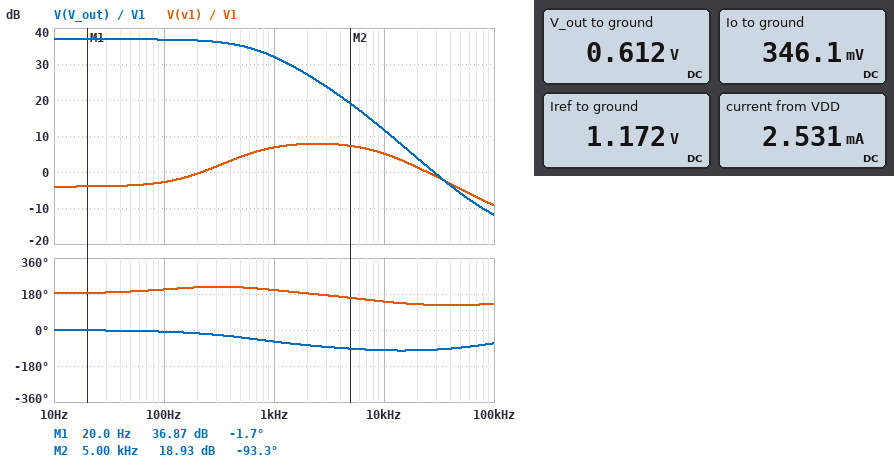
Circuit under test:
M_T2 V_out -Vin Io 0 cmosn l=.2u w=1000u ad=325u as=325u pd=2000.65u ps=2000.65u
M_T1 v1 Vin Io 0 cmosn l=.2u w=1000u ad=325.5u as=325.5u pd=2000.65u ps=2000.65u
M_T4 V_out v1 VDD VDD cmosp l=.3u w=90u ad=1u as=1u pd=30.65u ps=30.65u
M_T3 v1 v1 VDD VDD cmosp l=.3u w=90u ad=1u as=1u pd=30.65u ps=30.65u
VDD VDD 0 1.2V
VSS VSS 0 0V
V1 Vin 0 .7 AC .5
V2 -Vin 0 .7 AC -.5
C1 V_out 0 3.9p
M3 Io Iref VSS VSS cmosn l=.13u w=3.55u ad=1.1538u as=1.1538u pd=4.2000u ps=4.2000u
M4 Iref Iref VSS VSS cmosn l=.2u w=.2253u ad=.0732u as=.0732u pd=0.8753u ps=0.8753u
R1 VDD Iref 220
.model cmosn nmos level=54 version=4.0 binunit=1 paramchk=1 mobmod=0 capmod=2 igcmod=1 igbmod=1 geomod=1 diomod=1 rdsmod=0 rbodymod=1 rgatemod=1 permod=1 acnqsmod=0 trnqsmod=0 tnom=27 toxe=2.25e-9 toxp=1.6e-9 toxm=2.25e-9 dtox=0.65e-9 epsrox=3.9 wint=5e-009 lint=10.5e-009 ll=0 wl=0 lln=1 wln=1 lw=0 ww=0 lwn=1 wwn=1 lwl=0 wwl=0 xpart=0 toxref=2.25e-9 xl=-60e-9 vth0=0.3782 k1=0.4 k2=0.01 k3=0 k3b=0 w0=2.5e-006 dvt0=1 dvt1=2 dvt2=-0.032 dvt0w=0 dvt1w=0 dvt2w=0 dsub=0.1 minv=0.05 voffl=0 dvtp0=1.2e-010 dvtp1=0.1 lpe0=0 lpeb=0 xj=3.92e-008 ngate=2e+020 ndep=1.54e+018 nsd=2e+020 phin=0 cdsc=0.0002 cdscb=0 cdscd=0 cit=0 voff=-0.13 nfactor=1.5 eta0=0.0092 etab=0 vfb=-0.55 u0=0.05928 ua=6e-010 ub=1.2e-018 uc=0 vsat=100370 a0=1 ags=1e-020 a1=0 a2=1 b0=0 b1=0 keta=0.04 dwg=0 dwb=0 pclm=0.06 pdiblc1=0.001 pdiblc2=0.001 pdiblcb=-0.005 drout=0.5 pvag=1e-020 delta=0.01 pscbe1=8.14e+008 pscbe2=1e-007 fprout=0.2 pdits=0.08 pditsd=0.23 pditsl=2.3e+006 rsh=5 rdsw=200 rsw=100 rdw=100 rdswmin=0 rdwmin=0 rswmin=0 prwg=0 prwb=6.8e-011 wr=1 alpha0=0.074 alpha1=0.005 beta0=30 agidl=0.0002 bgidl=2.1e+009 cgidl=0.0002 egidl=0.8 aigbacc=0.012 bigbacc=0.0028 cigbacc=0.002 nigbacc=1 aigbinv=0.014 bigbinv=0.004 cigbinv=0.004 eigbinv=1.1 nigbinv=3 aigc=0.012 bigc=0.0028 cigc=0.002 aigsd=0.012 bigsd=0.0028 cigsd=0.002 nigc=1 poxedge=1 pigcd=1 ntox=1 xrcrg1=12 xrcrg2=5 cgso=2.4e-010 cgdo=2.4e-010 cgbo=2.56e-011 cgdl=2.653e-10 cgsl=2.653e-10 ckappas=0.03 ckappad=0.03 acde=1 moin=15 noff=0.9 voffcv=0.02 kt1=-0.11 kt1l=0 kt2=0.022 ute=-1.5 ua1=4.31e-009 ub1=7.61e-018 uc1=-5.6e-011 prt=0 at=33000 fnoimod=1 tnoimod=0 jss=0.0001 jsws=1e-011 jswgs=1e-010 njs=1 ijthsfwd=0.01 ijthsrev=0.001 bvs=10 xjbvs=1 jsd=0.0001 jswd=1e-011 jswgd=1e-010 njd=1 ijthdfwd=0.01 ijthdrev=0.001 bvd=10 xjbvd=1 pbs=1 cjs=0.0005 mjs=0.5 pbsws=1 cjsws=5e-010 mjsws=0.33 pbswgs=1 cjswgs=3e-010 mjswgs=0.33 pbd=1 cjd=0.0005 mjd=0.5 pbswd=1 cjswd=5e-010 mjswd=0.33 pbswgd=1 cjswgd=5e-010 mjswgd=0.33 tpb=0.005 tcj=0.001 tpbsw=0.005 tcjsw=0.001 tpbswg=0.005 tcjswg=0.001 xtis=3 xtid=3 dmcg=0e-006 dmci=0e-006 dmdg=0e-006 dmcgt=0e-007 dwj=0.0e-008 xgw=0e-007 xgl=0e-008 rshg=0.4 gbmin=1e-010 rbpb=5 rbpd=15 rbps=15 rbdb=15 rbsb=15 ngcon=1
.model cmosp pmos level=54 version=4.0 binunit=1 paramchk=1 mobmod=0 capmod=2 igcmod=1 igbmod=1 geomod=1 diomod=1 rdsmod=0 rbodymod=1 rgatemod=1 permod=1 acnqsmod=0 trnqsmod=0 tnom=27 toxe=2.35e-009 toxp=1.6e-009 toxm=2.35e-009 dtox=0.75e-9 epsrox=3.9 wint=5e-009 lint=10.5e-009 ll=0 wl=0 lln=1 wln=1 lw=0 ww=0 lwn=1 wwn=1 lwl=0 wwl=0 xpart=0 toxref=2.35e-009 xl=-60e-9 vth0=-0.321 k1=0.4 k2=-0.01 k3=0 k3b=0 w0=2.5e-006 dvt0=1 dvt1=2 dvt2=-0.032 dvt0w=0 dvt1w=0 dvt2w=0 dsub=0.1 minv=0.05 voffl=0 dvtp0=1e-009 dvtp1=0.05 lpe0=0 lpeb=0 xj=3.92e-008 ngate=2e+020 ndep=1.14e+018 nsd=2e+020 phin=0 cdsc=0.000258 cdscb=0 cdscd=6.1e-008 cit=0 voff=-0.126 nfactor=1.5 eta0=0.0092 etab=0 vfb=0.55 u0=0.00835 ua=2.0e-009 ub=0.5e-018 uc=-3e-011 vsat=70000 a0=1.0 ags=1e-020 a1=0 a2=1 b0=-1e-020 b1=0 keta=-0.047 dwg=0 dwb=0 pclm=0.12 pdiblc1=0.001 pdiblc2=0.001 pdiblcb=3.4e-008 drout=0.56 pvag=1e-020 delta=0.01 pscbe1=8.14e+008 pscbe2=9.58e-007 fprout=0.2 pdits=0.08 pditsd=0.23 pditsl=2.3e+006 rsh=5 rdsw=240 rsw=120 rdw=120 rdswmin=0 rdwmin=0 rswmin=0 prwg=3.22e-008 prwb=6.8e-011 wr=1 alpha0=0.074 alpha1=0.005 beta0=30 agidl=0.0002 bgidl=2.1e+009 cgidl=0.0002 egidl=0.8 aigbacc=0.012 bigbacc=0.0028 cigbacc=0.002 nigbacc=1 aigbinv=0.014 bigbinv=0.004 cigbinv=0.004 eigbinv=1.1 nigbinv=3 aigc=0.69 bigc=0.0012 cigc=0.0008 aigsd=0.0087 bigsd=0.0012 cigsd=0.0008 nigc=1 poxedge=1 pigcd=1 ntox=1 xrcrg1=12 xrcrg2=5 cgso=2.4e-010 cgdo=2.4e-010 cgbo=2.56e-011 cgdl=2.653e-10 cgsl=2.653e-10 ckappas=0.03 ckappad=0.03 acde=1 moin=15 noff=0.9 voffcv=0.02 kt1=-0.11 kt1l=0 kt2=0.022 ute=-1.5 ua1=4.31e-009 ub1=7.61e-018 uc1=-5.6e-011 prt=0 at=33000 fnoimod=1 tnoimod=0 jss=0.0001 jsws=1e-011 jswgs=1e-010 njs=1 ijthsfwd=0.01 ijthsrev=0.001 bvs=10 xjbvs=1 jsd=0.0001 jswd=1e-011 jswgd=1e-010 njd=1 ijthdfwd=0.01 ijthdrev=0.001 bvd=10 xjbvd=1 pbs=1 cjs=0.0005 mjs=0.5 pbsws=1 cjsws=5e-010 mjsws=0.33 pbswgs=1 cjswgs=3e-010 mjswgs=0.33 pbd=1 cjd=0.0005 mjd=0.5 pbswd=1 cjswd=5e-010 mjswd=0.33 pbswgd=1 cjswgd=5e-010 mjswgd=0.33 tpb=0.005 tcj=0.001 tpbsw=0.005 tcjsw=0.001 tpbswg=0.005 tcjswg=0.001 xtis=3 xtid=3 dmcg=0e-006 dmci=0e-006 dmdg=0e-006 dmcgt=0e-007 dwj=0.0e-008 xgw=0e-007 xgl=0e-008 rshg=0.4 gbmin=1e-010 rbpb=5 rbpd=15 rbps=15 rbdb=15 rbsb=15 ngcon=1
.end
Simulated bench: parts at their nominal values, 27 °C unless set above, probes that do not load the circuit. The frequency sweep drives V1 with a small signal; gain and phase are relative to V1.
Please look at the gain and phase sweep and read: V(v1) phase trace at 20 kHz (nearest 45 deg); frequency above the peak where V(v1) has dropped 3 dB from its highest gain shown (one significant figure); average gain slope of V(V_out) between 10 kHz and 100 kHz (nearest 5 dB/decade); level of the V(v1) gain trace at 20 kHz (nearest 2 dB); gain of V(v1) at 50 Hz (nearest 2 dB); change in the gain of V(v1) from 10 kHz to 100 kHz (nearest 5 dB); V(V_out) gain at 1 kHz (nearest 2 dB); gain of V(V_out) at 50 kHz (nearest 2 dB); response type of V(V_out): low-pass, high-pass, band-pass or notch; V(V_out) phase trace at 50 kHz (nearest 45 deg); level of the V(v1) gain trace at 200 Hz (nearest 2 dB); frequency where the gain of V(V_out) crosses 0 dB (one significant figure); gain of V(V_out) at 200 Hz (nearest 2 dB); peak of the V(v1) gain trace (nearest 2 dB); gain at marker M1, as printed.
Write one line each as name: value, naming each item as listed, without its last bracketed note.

V(v1) phase trace at 20 kHz: 135 deg
frequency above the peak where V(v1) has dropped 3 dB from its highest gain shown: 10 kHz
average gain slope of V(V_out) between 10 kHz and 100 kHz: -25 dB/decade
level of the V(v1) gain trace at 20 kHz: 2 dB
gain of V(v1) at 50 Hz: -4 dB
change in the gain of V(v1) from 10 kHz to 100 kHz: -15 dB
V(V_out) gain at 1 kHz: 32 dB
gain of V(V_out) at 50 kHz: -6 dB
response type of V(V_out): low-pass, high-pass, band-pass or notch: low-pass
V(V_out) phase trace at 50 kHz: -90 deg
level of the V(v1) gain trace at 200 Hz: 0 dB
frequency where the gain of V(V_out) crosses 0 dB: 30 kHz
gain of V(V_out) at 200 Hz: 36 dB
peak of the V(v1) gain trace: 8 dB
gain at marker M1, as printed: 36.87 dB
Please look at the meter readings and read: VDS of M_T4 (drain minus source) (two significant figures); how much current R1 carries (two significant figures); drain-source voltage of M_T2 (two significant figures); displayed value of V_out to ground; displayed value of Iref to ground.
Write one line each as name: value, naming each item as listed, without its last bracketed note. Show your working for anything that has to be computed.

VDS of M_T4 (drain minus source): 612 mV - 1.2 V = -590 mV
how much current R1 carries: (1.2 V - 1.172 V) / 220 Ω = 130 µA
drain-source voltage of M_T2: 612 mV - 346.1 mV = 270 mV
displayed value of V_out to ground: 0.612 V
displayed value of Iref to ground: 1.172 V
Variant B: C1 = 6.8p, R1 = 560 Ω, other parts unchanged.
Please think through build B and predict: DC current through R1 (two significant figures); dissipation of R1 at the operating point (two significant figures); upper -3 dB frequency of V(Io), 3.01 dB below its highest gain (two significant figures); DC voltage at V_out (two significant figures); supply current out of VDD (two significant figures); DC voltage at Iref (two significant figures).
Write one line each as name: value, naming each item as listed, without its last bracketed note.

DC current through R1: 120 µA
dissipation of R1 at the operating point: 8.1 µW
upper -3 dB frequency of V(Io), 3.01 dB below its highest gain: 720 Hz
DC voltage at V_out: 620 mV
supply current out of VDD: 2.4 mA
DC voltage at Iref: 1.1 V
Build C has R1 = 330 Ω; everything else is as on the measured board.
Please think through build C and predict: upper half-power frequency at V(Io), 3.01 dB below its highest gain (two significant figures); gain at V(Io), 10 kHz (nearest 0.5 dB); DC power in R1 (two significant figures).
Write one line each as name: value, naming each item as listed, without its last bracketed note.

upper half-power frequency at V(Io), 3.01 dB below its highest gain: 730 Hz
gain at V(Io), 10 kHz: -15.0 dB
DC power in R1: 5.2 µW
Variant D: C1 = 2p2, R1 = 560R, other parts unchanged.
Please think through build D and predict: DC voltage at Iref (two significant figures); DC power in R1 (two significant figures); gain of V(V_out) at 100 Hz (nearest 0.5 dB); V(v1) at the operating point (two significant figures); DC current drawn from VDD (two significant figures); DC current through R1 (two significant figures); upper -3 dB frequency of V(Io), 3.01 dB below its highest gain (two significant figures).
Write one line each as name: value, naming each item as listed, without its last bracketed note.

DC voltage at Iref: 1.1 V
DC power in R1: 8.1 µW
gain of V(V_out) at 100 Hz: 37.0 dB
V(v1) at the operating point: 620 mV
DC current drawn from VDD: 2.4 mA
DC current through R1: 120 µA
upper -3 dB frequency of V(Io), 3.01 dB below its highest gain: 720 Hz
